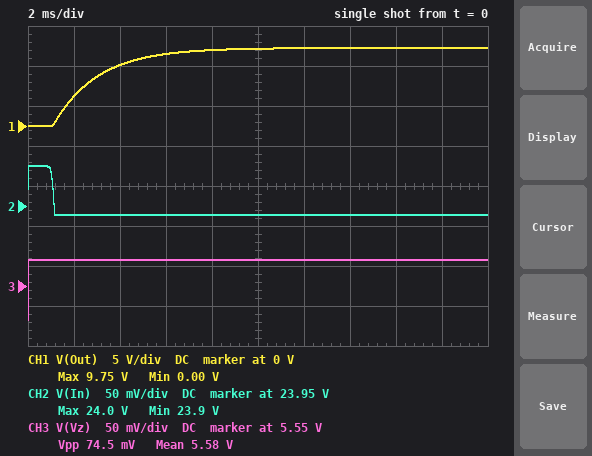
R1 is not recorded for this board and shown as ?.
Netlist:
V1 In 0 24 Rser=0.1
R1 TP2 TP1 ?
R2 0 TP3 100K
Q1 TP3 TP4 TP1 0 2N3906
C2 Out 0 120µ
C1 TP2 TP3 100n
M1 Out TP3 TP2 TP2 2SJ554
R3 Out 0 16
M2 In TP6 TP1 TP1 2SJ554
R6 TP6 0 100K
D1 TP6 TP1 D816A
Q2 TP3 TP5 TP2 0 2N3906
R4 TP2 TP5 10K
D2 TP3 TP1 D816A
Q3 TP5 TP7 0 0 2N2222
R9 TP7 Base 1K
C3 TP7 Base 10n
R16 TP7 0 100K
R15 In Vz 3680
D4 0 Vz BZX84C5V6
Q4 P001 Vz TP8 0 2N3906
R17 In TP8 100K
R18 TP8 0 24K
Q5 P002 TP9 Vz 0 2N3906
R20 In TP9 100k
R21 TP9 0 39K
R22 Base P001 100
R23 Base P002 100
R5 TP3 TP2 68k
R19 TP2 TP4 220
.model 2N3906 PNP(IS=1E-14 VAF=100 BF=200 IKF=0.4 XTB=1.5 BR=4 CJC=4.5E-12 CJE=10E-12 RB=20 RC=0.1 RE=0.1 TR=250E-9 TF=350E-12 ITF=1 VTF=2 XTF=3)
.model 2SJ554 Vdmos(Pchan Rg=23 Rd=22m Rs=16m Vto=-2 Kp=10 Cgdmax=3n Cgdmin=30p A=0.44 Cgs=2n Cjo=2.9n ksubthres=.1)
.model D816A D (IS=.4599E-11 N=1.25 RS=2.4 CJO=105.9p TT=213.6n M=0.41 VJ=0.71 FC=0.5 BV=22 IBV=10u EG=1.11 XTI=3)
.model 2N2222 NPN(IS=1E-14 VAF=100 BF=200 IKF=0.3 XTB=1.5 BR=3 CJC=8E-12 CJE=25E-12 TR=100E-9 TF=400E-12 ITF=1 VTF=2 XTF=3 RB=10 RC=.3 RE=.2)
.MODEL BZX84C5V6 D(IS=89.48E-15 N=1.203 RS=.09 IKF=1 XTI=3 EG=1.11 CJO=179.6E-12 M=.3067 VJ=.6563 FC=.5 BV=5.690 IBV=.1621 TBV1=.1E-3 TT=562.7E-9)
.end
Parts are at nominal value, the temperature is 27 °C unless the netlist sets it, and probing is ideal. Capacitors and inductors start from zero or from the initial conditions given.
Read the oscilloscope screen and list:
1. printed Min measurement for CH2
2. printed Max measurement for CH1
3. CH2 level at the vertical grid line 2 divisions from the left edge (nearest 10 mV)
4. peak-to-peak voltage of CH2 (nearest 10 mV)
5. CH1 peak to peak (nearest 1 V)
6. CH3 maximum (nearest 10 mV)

23.9 V
9.75 V
23.94 V
60 mV
10 V
5.58 V
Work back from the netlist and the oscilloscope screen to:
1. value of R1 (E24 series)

1 Ω
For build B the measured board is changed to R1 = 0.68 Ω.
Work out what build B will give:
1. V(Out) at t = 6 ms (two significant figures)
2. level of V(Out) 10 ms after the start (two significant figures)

13 V
14 V
